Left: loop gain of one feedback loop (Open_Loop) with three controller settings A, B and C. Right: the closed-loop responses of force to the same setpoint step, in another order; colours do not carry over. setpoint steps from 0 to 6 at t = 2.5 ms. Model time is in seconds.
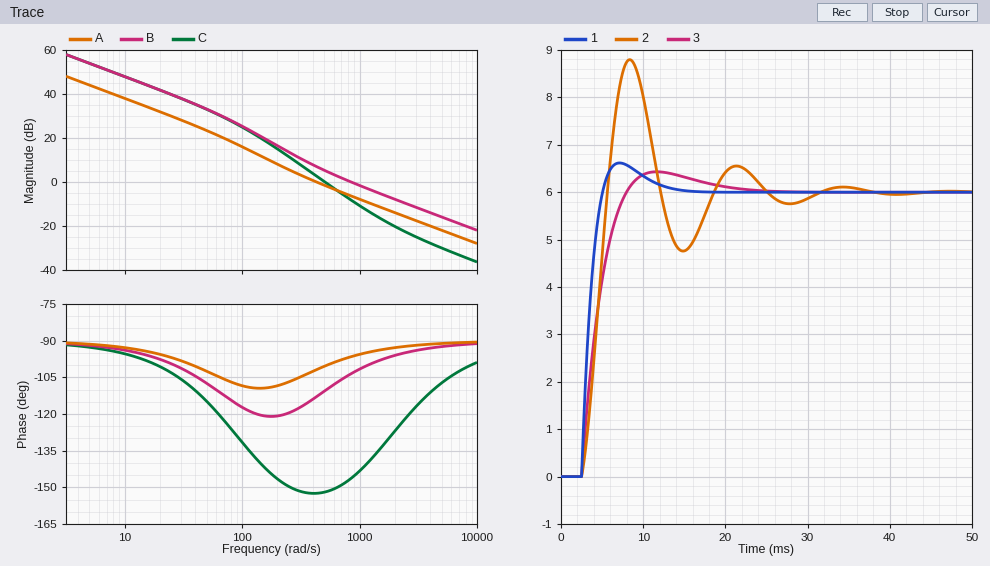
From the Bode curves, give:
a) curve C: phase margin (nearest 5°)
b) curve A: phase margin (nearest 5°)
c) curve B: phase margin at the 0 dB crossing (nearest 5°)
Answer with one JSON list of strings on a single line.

["30°", "80°", "75°"]
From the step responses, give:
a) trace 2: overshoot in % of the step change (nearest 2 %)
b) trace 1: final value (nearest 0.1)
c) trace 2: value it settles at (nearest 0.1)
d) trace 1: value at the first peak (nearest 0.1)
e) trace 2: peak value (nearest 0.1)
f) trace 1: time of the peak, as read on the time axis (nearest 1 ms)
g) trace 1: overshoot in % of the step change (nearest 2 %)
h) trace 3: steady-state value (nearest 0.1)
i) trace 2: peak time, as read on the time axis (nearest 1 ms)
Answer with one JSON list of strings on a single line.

["46 %", "6.0", "6.0", "6.6", "8.8", "7 ms", "10 %", "6.0", "8 ms"]
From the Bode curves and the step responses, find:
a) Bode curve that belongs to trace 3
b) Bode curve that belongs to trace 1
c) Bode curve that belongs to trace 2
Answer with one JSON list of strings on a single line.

["A", "B", "C"]
